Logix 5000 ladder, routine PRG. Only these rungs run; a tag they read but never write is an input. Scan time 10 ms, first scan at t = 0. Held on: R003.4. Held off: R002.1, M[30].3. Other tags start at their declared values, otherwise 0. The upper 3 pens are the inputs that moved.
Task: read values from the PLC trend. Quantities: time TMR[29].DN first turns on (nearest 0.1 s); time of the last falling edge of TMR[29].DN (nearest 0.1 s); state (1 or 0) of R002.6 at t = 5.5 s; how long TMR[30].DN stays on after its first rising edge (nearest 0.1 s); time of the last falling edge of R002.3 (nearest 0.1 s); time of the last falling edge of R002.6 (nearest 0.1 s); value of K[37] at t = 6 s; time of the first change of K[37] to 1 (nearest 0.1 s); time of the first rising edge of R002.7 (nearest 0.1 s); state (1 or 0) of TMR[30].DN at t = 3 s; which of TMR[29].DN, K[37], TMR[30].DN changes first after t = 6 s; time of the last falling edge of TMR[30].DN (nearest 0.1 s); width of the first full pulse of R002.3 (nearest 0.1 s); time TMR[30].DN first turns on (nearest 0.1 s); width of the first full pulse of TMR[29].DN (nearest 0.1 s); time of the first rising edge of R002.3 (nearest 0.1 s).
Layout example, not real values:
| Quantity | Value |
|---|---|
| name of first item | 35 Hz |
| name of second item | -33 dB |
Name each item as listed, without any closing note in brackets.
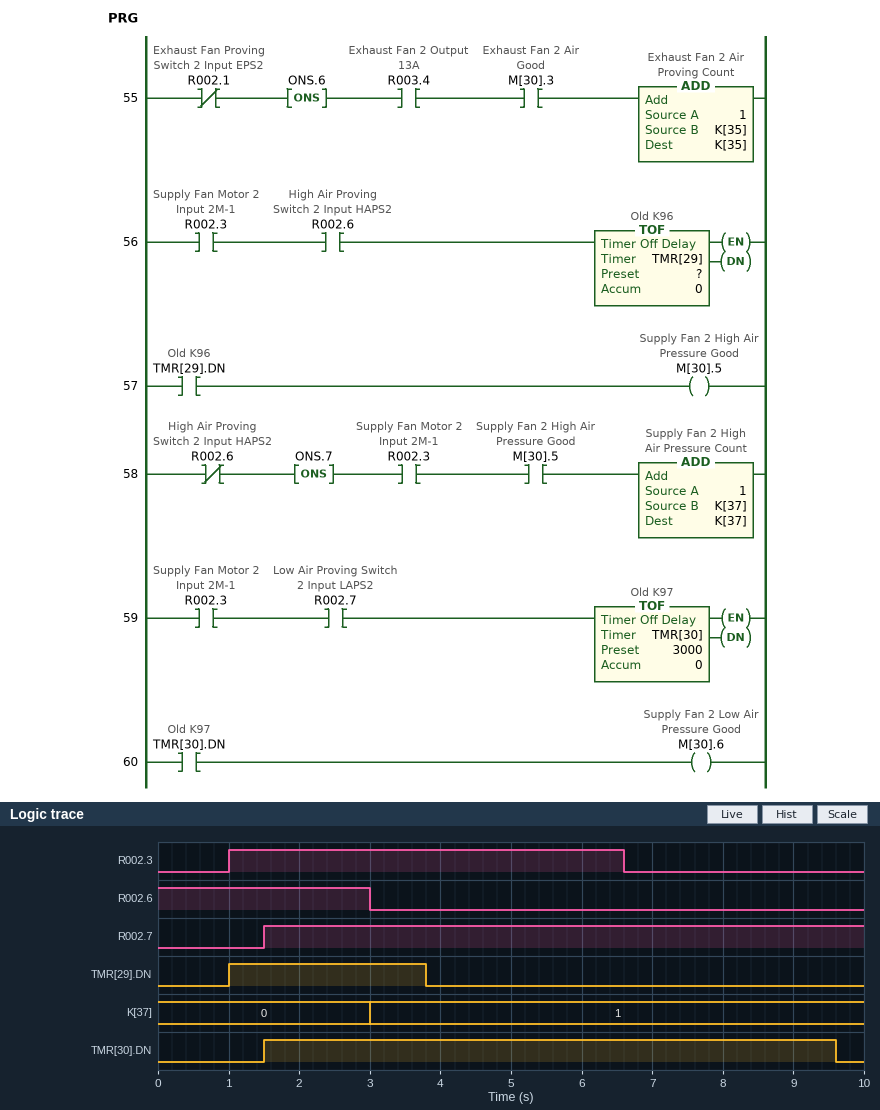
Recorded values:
| Quantity | Value |
|---|---|
| time TMR[29].DN first turns on | 1.0 s |
| time of the last falling edge of TMR[29].DN | 3.8 s |
| state (1 or 0) of R002.6 at t = 5.5 s | 0 |
| how long TMR[30].DN stays on after its first rising edge | 8.1 s |
| time of the last falling edge of R002.3 | 6.6 s |
| time of the last falling edge of R002.6 | 3.0 s |
| value of K[37] at t = 6 s | 1 |
| time of the first change of K[37] to 1 | 3.0 s |
| time of the first rising edge of R002.7 | 1.5 s |
| state (1 or 0) of TMR[30].DN at t = 3 s | 1 |
| which of TMR[29].DN, K[37], TMR[30].DN changes first after t = 6 s | TMR[30].DN |
| time of the last falling edge of TMR[30].DN | 9.6 s |
| width of the first full pulse of R002.3 | 5.6 s |
| time TMR[30].DN first turns on | 1.5 s |
| width of the first full pulse of TMR[29].DN | 2.8 s |
| time of the first rising edge of R002.3 | 1.0 s |
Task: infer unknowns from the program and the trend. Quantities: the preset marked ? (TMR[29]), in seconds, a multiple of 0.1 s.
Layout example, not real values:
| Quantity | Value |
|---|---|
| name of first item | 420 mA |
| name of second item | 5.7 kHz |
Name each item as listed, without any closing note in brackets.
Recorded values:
| Quantity | Value |
|---|---|
| the preset marked ? (TMR[29]), in seconds, a multiple of 0.1 s | 0.8 s |
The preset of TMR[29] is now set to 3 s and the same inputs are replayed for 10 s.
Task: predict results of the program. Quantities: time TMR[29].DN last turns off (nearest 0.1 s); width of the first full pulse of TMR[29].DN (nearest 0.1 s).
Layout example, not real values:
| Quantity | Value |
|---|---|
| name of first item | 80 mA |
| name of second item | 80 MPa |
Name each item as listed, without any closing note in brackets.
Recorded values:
| Quantity | Value |
|---|---|
| time TMR[29].DN last turns off | 6.0 s |
| width of the first full pulse of TMR[29].DN | 5.0 s |
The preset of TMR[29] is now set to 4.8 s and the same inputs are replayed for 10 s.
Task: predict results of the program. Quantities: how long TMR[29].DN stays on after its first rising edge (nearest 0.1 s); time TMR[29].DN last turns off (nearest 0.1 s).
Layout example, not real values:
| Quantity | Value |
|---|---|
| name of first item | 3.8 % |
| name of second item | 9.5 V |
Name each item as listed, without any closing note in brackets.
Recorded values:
| Quantity | Value |
|---|---|
| how long TMR[29].DN stays on after its first rising edge | 6.8 s |
| time TMR[29].DN last turns off | 7.8 s |
